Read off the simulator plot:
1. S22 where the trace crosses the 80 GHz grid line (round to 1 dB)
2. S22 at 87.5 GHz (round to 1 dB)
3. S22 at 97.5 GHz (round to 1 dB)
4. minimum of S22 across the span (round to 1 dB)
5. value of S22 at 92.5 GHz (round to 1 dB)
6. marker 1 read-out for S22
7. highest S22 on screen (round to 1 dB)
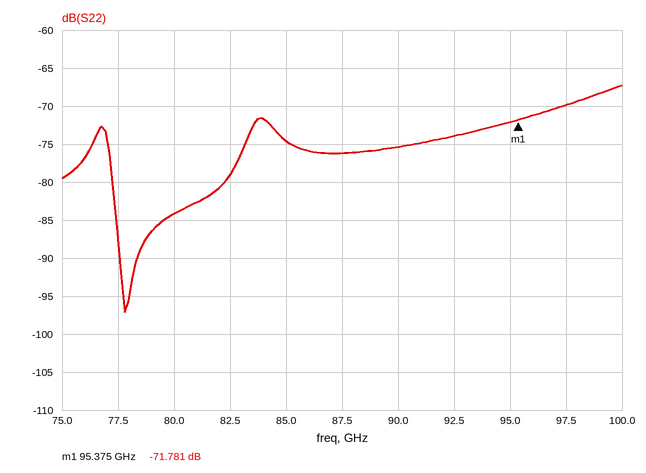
-84 dB
-76 dB
-70 dB
-97 dB
-74 dB
-71.781 dB
-67 dB
